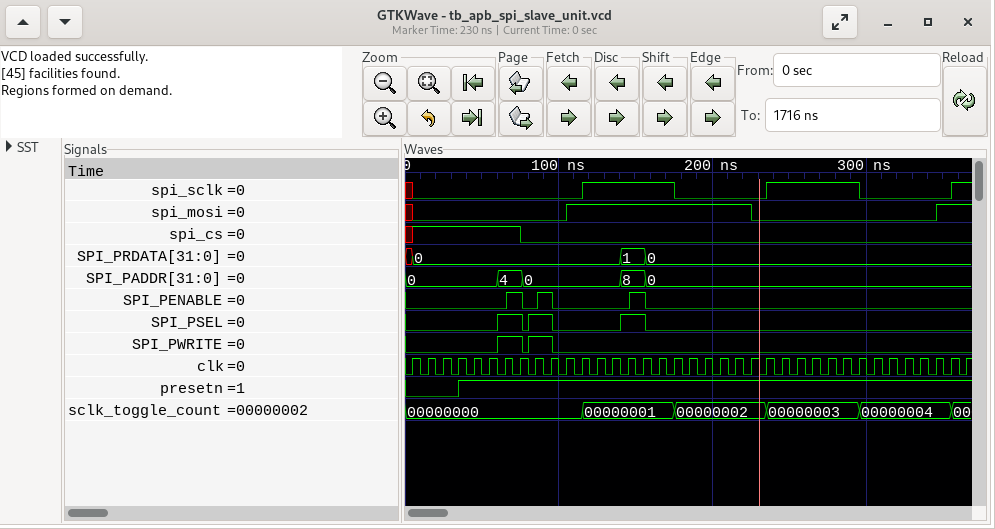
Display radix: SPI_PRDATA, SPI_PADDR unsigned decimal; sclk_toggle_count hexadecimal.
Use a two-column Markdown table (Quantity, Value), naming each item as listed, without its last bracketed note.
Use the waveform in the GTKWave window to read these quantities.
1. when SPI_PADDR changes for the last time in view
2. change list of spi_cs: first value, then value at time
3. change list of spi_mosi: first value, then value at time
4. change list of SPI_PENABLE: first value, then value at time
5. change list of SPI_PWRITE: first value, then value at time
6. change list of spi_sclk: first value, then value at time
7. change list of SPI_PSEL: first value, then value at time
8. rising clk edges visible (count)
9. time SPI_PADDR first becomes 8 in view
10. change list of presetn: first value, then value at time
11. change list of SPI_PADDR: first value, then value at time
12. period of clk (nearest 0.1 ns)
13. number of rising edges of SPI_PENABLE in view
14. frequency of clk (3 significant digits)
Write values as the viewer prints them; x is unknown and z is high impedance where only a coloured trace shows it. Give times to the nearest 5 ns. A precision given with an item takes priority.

| Quantity | Value |
|---|---|
| when SPI_PADDR changes for the last time in view | 155 ns |
| change list of spi_cs: first value, then value at time | x, 1 at 5 ns, 0 at 75 ns |
| change list of spi_mosi: first value, then value at time | x, 0 at 5 ns, 1 at 105 ns, 0 at 225 ns, 1 at 345 ns |
| change list of SPI_PENABLE: first value, then value at time | 0, 1 at 65 ns, 0 at 75 ns, 1 at 85 ns, 0 at 95 ns, 1 at 145 ns, 0 at 155 ns |
| change list of SPI_PWRITE: first value, then value at time | 0, 1 at 60 ns, 0 at 75 ns, 1 at 80 ns, 0 at 95 ns |
| change list of spi_sclk: first value, then value at time | x, 0 at 5 ns, 1 at 115 ns, 0 at 175 ns, 1 at 235 ns, 0 at 295 ns, 1 at 355 ns |
| change list of SPI_PSEL: first value, then value at time | 0, 1 at 60 ns, 0 at 75 ns, 1 at 80 ns, 0 at 95 ns, 1 at 140 ns, 0 at 155 ns |
| rising clk edges visible | 37 |
| time SPI_PADDR first becomes 8 in view | 140 ns |
| change list of presetn: first value, then value at time | 0, 1 at 35 ns |
| change list of SPI_PADDR: first value, then value at time | 0, 4 at 60 ns, 0 at 75 ns, 8 at 140 ns, 0 at 155 ns |
| period of clk | 10 ns |
| number of rising edges of SPI_PENABLE in view | 3 |
| frequency of clk | 100 MHz |
